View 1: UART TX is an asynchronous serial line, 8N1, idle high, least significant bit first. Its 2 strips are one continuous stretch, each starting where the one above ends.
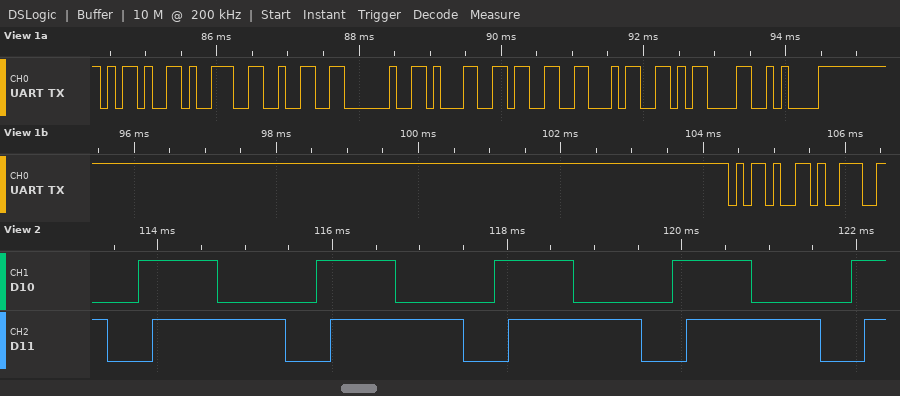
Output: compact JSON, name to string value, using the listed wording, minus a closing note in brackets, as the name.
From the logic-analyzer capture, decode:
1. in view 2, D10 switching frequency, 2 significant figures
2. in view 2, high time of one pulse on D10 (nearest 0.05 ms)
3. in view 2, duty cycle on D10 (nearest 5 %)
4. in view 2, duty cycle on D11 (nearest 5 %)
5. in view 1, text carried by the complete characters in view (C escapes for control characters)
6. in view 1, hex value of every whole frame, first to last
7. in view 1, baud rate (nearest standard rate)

{"in view 2, D10 switching frequency, 2 significant figures": "490 Hz", "in view 2, high time of one pulse on D10": "0.90 ms", "in view 2, duty cycle on D10": "45 %", "in view 2, duty cycle on D11": "75 %", "in view 1, text carried by the complete characters in view": "\"-92 134\\r\\n-9\"", "in view 1, hex value of every whole frame, first to last": "2D 39 32 20 31 33 34 0D 0A 2D 39", "in view 1, baud rate": "9600 baud"}
